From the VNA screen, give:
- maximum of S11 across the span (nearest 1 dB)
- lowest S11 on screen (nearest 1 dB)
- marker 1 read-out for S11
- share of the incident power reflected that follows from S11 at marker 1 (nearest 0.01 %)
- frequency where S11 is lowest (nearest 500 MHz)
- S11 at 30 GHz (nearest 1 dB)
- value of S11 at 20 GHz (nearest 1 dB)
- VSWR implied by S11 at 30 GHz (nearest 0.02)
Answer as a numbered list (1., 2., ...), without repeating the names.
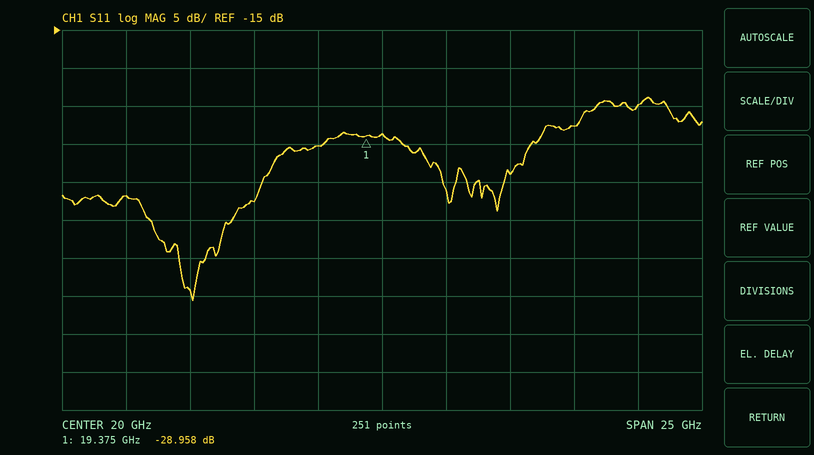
1. -24 dB
2. -51 dB
3. -28.958 dB
4. 0.13 %
5. 12.5 GHz
6. -25 dB
7. -29 dB
8. 1.12
